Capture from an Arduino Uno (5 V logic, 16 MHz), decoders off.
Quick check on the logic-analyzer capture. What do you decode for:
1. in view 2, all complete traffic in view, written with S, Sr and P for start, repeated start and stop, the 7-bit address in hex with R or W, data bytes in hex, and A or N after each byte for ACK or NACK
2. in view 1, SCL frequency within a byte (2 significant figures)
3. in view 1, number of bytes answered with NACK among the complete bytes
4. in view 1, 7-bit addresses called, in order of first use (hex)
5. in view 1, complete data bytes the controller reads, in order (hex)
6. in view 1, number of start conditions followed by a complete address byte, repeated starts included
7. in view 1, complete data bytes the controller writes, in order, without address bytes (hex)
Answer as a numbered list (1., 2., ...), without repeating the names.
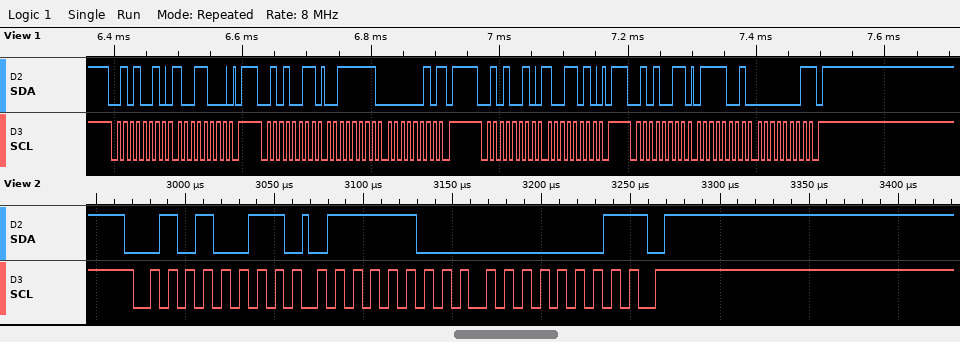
1. S 29R A 7C A 01 N P
2. 100 kHz
3. 2
4. 0x29
5. 3F 02 79 01
6. 4
7. 98 9A
